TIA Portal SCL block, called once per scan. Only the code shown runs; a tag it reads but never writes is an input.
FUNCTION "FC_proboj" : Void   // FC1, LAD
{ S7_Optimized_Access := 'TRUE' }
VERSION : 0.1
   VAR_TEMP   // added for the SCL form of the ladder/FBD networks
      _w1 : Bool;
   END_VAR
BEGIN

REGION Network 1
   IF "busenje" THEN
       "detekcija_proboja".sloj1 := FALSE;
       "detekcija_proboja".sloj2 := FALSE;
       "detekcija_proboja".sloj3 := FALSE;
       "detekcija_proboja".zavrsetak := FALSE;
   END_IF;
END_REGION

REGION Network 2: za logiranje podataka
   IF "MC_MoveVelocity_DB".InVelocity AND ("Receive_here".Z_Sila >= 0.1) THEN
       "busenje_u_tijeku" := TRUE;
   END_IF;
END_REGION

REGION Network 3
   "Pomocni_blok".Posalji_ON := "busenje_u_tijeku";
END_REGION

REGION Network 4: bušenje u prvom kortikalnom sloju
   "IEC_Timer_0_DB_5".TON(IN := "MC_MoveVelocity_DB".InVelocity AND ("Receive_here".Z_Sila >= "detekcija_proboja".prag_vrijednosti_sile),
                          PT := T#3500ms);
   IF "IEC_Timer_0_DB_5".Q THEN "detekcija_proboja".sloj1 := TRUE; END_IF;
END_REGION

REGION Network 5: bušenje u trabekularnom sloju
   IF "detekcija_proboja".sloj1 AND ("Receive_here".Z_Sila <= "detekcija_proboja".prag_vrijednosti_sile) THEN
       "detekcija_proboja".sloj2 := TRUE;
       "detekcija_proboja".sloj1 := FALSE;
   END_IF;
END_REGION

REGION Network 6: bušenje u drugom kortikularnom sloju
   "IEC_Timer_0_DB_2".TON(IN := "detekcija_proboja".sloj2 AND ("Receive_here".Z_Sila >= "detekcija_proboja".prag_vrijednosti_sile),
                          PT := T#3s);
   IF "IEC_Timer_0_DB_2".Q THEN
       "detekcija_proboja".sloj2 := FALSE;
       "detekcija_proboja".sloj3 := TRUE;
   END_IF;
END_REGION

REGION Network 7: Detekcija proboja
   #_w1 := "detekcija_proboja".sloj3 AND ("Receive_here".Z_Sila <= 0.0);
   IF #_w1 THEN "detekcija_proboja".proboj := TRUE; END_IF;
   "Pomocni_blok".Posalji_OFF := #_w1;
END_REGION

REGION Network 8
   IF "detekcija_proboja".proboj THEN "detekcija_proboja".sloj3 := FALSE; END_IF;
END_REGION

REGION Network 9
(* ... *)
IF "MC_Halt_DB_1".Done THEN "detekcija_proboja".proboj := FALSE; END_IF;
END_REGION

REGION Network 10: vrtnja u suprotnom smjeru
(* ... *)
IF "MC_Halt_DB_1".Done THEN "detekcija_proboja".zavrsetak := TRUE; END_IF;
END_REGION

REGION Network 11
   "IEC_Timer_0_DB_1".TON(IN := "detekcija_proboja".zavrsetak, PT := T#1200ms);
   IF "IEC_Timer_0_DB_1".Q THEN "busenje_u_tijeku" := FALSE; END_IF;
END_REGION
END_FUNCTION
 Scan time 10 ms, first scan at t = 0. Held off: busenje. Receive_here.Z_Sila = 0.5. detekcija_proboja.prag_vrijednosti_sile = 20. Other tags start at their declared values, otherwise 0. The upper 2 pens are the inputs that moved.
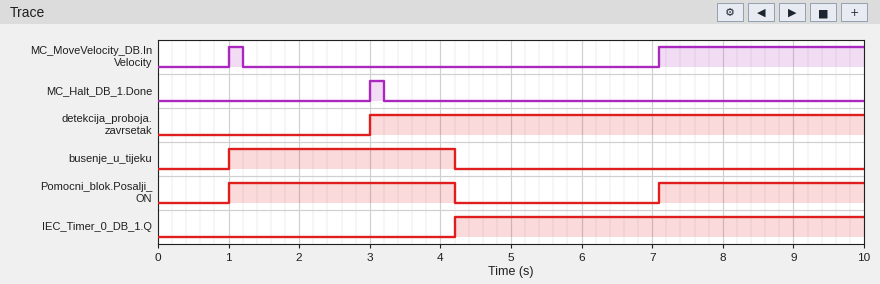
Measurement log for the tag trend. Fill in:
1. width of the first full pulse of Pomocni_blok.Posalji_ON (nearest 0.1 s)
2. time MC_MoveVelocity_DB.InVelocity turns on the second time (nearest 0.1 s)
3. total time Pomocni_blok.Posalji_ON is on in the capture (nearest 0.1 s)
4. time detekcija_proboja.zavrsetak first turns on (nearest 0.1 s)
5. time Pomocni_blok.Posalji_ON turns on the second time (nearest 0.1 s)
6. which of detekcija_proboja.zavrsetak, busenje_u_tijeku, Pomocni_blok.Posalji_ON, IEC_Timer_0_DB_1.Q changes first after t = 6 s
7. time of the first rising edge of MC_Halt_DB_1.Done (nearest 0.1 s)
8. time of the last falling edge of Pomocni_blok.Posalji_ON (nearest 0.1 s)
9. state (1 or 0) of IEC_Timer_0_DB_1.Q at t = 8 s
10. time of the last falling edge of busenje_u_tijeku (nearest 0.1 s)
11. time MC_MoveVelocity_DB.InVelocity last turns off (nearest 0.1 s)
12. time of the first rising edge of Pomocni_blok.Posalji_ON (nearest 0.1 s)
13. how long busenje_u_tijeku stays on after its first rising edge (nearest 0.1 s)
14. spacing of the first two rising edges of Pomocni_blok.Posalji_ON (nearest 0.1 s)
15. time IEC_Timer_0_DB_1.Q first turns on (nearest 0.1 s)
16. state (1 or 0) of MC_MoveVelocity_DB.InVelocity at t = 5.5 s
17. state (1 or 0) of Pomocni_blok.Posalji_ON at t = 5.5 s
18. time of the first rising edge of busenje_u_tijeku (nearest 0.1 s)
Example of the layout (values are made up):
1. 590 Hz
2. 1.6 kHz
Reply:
1. 3.2 s
2. 7.1 s
3. 6.1 s
4. 3.0 s
5. 7.1 s
6. Pomocni_blok.Posalji_ON
7. 3.0 s
8. 4.2 s
9. 1
10. 4.2 s
11. 1.2 s
12. 1.0 s
13. 3.2 s
14. 6.1 s
15. 4.2 s
16. 0
17. 0
18. 1.0 s
